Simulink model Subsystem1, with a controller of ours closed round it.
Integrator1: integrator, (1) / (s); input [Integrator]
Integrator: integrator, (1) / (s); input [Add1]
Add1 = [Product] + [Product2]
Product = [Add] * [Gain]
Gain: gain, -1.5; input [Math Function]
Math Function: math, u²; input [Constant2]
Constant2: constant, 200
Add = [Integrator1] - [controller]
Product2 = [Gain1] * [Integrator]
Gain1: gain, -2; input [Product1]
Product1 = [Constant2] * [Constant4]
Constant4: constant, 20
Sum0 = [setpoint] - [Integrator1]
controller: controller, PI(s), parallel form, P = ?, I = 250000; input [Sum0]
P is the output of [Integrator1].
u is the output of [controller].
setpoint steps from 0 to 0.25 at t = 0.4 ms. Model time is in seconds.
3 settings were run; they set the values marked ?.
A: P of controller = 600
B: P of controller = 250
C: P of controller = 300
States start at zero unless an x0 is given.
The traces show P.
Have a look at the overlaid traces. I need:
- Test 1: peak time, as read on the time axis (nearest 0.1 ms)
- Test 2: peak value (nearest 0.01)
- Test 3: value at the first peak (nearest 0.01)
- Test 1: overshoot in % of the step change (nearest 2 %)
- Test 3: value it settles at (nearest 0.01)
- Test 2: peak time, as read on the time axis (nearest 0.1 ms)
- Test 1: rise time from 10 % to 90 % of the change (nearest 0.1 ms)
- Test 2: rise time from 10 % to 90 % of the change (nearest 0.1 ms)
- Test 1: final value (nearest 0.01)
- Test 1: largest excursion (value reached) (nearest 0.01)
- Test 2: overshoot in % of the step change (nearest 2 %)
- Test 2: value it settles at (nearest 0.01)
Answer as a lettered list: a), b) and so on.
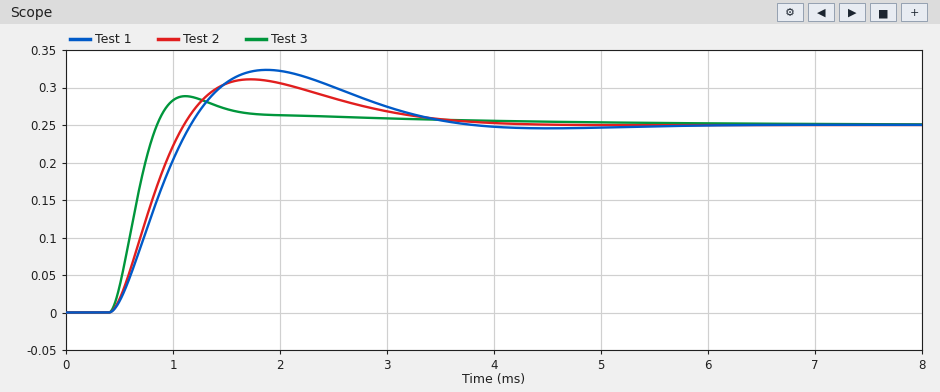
a) 1.9 ms
b) 0.31
c) 0.29
d) 30 %
e) 0.25
f) 1.7 ms
g) 0.5 ms
h) 0.5 ms
i) 0.25
j) 0.32
k) 24 %
l) 0.25
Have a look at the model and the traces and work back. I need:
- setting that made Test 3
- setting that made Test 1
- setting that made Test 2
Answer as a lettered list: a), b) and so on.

a) A
b) B
c) C
